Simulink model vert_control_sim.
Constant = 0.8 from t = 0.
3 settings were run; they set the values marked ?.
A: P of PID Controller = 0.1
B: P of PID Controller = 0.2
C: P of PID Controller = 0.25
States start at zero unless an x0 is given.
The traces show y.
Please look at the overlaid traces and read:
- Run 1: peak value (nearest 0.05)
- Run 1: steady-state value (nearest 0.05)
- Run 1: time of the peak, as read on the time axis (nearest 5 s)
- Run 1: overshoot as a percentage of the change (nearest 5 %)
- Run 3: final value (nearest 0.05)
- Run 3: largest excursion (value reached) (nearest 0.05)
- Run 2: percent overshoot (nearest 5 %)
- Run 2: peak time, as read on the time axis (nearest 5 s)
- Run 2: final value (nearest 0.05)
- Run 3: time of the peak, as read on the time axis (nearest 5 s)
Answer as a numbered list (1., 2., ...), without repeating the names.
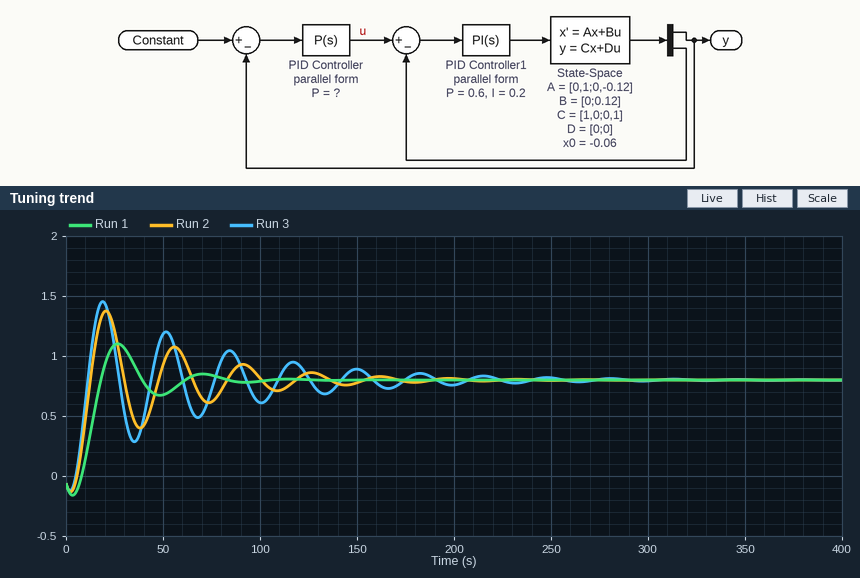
1. 1.10
2. 0.80
3. 25 s
4. 35 %
5. 0.80
6. 1.45
7. 65 %
8. 20 s
9. 0.80
10. 20 s
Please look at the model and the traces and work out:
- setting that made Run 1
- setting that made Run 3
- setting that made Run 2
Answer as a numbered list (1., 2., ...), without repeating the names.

1. A
2. C
3. B
